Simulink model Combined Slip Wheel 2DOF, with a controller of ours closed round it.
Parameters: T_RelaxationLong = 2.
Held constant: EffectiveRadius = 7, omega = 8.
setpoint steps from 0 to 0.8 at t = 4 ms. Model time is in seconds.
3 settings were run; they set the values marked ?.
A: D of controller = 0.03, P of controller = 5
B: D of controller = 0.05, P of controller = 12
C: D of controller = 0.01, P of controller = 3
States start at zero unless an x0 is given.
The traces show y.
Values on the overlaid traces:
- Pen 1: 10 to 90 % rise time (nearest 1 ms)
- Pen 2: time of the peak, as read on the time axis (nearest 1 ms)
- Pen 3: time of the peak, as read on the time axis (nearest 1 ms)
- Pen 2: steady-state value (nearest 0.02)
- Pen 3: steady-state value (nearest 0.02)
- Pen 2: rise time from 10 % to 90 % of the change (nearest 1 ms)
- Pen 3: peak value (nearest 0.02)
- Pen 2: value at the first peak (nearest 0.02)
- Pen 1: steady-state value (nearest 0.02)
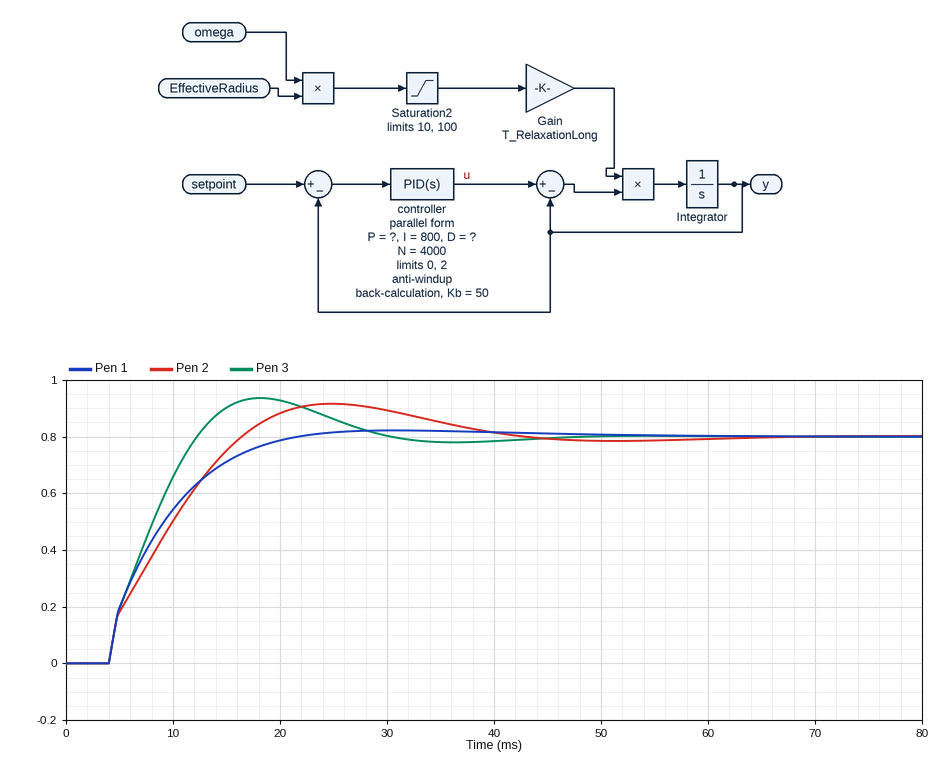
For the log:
11 ms
25 ms
18 ms
0.80
0.80
10 ms
0.94
0.92
0.80
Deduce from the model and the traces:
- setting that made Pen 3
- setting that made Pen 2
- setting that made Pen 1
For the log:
C
A
B
